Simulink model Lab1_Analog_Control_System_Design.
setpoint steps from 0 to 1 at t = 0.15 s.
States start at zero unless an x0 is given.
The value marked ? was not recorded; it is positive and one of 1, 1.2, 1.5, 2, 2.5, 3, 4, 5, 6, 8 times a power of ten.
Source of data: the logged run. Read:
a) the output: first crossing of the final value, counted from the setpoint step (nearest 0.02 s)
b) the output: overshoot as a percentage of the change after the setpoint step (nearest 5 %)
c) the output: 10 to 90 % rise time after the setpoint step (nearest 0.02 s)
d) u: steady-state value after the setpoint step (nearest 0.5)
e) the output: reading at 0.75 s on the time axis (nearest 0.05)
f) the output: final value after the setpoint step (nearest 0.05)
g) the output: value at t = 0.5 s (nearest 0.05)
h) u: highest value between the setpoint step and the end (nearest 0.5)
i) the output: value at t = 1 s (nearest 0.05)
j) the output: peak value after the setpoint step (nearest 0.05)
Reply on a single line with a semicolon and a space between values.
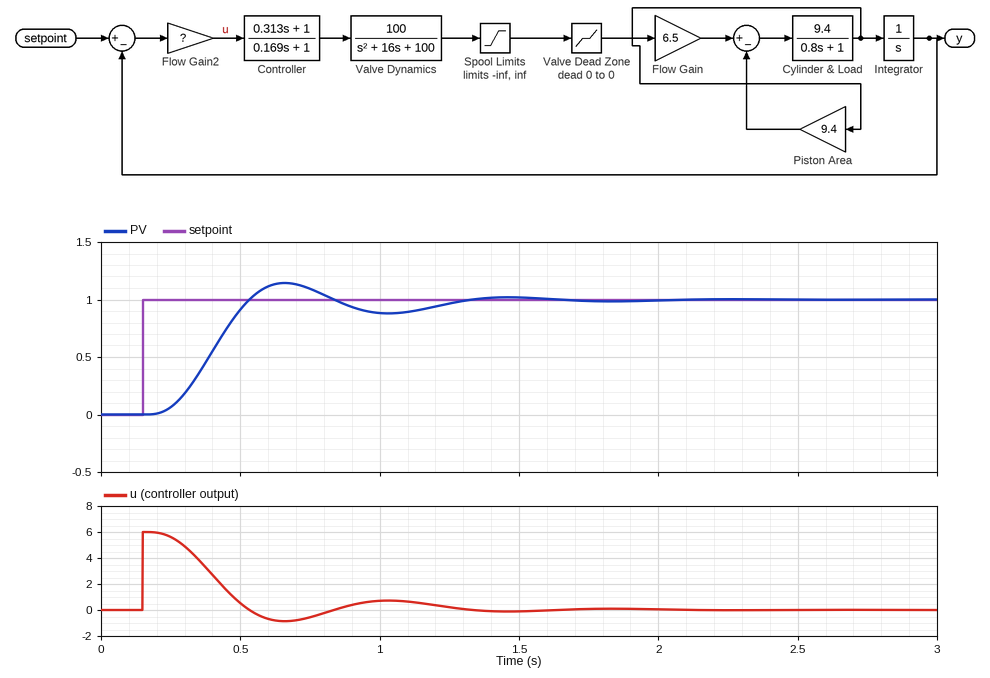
0.38 s; 15 %; 0.22 s; 0.0; 1.10; 1.00; 0.90; 6.0; 0.90; 1.15
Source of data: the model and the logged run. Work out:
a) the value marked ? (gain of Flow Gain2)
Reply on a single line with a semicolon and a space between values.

6
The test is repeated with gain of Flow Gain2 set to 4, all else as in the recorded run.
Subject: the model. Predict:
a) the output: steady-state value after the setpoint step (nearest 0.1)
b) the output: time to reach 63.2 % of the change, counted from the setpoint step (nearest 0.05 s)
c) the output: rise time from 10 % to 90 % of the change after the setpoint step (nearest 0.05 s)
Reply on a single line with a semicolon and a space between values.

1.0; 0.35 s; 0.35 s
